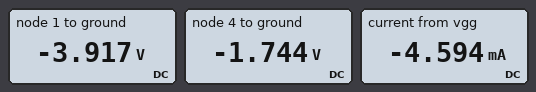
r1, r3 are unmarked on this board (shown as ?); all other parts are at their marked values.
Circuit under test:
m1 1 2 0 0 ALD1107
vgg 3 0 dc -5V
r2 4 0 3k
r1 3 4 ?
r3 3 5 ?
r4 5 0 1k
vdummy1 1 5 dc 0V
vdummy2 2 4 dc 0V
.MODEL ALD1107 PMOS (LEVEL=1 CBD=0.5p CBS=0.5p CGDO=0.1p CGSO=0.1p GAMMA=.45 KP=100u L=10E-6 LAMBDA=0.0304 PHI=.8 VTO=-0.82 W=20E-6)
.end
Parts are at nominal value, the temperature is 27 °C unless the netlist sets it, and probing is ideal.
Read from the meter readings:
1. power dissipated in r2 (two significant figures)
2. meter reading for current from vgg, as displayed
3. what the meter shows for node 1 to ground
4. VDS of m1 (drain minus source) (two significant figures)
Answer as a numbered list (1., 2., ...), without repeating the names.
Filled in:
1. 1.0 mW
2. -4.594 mA
3. -3.917 V
4. -3.9 V
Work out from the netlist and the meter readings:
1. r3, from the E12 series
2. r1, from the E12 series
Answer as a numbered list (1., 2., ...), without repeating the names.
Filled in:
1. 270 Ω
2. 5.6 kΩ
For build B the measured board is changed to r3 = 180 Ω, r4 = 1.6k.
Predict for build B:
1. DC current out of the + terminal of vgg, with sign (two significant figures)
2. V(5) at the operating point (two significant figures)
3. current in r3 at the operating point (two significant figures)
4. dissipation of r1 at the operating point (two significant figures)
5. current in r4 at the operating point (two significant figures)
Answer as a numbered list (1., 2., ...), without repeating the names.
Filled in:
1. -3.5 mA
2. -4.5 V
3. 2.9 mA
4. 1.9 mW
5. 2.8 mA
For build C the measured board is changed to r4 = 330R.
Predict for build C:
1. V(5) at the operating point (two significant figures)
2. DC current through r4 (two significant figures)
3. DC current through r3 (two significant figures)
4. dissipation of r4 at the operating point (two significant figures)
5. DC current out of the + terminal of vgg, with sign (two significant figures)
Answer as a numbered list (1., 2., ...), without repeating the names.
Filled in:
1. -2.7 V
2. 8.3 mA
3. 8.4 mA
4. 23 mW
5. -9.0 mA
